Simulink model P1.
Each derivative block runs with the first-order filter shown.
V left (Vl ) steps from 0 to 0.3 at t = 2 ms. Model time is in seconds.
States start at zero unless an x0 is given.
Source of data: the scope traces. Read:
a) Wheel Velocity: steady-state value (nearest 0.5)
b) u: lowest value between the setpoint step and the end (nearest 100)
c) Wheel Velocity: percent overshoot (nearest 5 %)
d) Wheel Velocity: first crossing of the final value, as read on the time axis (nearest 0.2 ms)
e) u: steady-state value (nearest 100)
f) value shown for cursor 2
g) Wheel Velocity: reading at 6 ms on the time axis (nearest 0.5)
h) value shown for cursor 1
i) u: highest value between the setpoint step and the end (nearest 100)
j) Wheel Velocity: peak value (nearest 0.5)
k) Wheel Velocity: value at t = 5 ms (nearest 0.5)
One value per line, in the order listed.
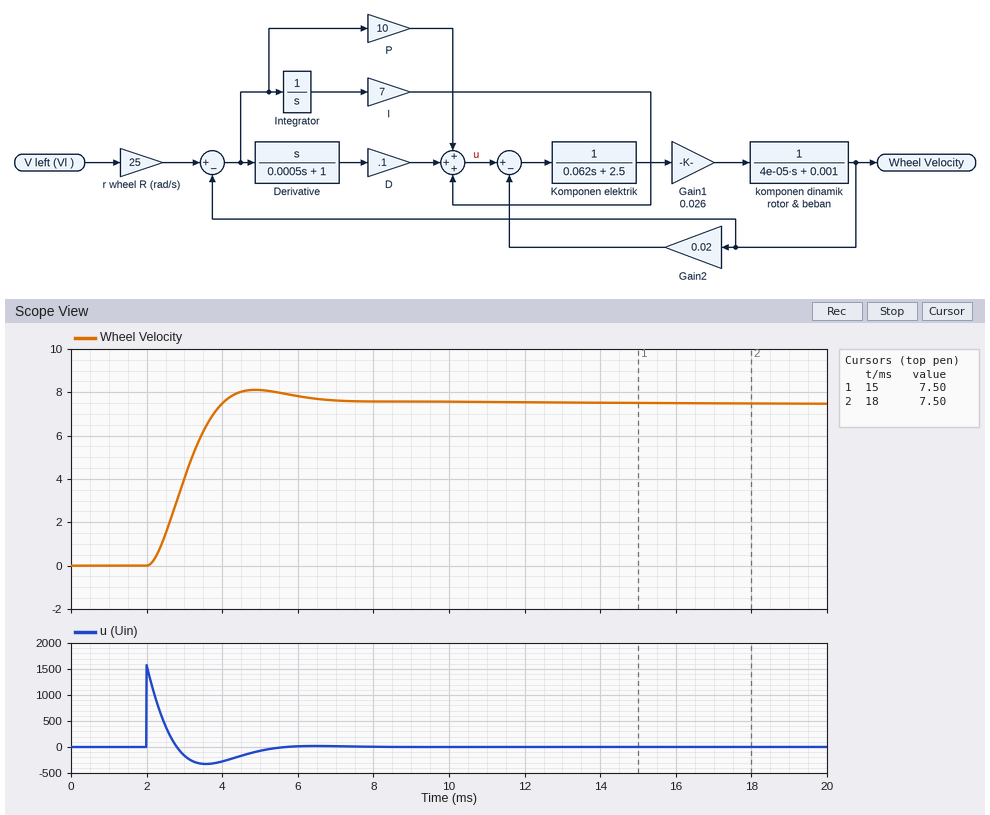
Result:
7.5
-300
10 %
4.0 ms
0
7.50
8.0
7.50
1600
8.0
8.0
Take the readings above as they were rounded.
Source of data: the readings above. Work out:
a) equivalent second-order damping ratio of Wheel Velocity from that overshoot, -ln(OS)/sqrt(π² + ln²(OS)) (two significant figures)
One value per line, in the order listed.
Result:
0.59
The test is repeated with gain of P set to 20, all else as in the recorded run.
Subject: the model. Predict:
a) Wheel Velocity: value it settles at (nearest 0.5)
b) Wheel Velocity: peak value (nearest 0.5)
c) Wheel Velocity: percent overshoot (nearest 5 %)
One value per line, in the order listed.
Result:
7.5
8.5
15 %
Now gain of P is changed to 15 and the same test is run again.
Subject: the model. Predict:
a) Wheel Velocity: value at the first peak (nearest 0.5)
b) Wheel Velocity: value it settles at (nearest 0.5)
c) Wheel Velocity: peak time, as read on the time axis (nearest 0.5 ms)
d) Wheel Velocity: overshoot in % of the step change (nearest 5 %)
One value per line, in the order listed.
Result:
8.5
7.5
5.0 ms
15 %
